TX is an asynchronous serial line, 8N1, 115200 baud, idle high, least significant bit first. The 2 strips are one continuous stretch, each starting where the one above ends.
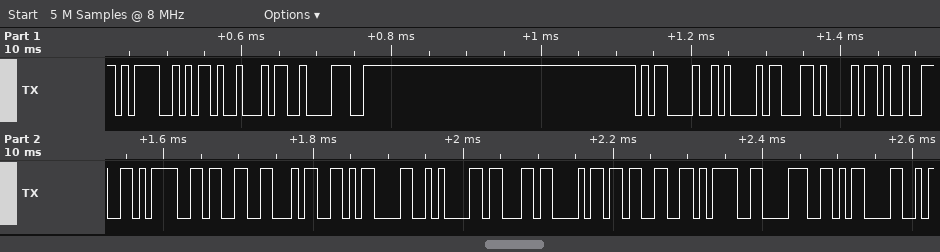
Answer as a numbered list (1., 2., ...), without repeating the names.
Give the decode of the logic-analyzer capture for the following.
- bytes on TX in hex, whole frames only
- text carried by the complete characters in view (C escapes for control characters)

1. 3D 2D 34 38 0D 0A 63 68 32 3D 33 34 0D 0A 63 68 33 3D 38 0D
2. "=-48\r\nch2=34\r\nch3=8\r"
